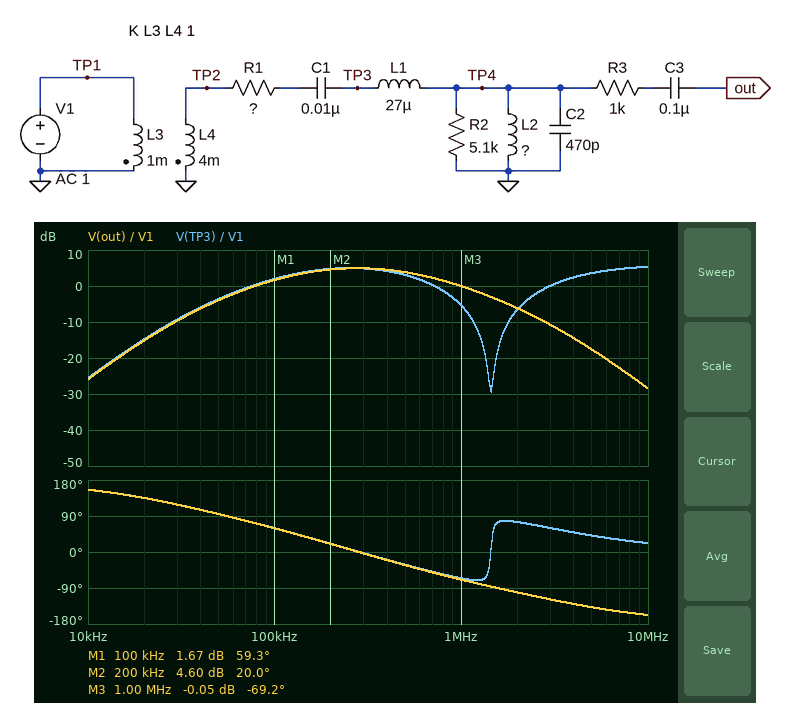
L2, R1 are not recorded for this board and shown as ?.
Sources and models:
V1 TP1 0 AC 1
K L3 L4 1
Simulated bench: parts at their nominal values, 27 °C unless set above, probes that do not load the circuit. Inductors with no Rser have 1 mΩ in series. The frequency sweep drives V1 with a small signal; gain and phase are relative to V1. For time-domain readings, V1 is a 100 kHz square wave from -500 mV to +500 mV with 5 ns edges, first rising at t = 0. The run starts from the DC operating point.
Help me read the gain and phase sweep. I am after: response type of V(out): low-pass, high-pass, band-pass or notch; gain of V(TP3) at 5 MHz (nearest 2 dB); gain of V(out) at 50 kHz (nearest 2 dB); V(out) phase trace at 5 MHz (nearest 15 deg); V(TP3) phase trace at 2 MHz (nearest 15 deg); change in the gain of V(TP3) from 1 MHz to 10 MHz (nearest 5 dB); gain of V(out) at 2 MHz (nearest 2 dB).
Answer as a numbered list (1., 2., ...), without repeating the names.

1. band-pass
2. 4 dB
3. -4 dB
4. -135 deg
5. 75 deg
6. 10 dB
7. -6 dB
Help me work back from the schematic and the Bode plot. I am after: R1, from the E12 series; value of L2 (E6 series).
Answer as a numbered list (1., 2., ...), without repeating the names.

1. 680 Ω
2. 680 µH
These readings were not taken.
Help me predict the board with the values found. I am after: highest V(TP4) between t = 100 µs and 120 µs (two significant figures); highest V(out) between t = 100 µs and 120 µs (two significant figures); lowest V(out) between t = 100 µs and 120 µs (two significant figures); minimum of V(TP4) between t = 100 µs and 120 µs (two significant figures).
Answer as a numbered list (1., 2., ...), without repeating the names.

1. 1.4 V
2. 1.4 V
3. -1.4 V
4. -1.4 V
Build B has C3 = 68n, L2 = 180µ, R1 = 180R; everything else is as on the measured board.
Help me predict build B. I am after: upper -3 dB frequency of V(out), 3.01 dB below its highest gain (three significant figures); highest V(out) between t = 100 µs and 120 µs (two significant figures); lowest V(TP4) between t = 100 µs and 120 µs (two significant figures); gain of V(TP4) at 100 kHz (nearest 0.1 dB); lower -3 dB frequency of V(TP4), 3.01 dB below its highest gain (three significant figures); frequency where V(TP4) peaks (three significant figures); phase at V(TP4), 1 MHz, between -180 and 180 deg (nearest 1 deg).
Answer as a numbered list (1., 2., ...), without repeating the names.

1. 1.80 MHz
2. 2.2 V
3. -2.2 V
4. 2.1 dB
5. 614 kHz
6. 1.35 MHz
7. -29 deg
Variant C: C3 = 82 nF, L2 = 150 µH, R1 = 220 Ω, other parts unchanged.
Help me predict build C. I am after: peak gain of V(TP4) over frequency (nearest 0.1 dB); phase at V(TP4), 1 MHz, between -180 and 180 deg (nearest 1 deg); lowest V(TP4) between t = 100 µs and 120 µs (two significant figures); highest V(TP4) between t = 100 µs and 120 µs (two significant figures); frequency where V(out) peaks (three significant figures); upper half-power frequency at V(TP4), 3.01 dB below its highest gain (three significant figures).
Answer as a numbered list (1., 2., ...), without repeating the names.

1. 7.8 dB
2. -31 deg
3. -1.9 V
4. 1.9 V
5. 1.27 MHz
6. 1.80 MHz
